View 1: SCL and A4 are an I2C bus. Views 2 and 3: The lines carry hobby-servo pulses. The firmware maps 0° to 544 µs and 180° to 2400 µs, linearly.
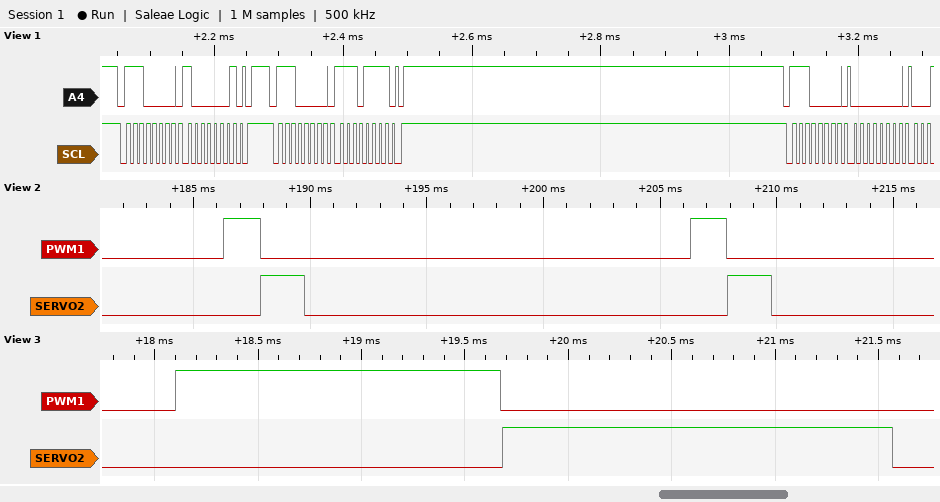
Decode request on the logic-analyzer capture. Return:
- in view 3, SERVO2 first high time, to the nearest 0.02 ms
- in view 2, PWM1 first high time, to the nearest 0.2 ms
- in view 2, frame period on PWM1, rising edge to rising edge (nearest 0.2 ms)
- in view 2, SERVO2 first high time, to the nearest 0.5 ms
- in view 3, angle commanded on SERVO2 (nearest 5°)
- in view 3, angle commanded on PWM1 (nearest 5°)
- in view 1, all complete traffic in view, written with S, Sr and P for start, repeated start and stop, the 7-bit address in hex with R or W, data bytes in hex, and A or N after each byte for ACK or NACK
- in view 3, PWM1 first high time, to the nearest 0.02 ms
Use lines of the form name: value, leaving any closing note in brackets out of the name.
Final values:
in view 3, SERVO2 first high time, to the nearest 0.02 ms: 1.88 ms
in view 2, PWM1 first high time, to the nearest 0.2 ms: 1.6 ms
in view 2, frame period on PWM1, rising edge to rising edge: 20.0 ms
in view 2, SERVO2 first high time, to the nearest 0.5 ms: 2.0 ms
in view 3, angle commanded on SERVO2: 130°
in view 3, angle commanded on PWM1: 100°
in view 1, all complete traffic in view, written with S, Sr and P for start, repeated start and stop, the 7-bit address in hex with R or W, data bytes in hex, and A or N after each byte for ACK or NACK: S 70W A 81 A P S 70W A EF A P S 70W A 00 A
in view 3, PWM1 first high time, to the nearest 0.02 ms: 1.58 ms
